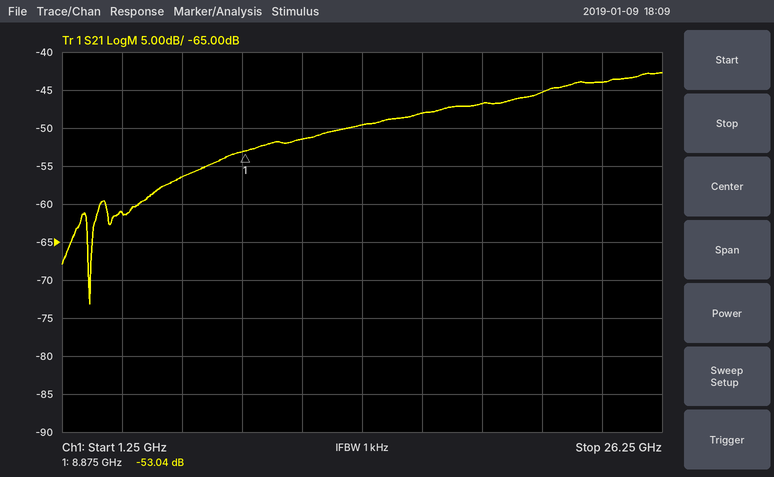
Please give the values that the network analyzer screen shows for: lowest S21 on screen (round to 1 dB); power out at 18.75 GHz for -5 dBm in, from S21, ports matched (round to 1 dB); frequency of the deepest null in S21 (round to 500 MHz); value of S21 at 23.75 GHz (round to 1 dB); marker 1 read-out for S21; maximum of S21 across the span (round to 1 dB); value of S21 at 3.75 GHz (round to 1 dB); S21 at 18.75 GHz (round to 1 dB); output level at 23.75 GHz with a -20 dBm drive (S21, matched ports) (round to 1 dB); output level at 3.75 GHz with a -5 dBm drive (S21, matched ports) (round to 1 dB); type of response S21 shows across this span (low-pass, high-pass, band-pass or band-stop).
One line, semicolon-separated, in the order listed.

-73 dB; -52 dBm; 2.5 GHz; -44 dB; -53.04 dB; -43 dB; -61 dB; -47 dB; -64 dBm; -66 dBm; high-pass
